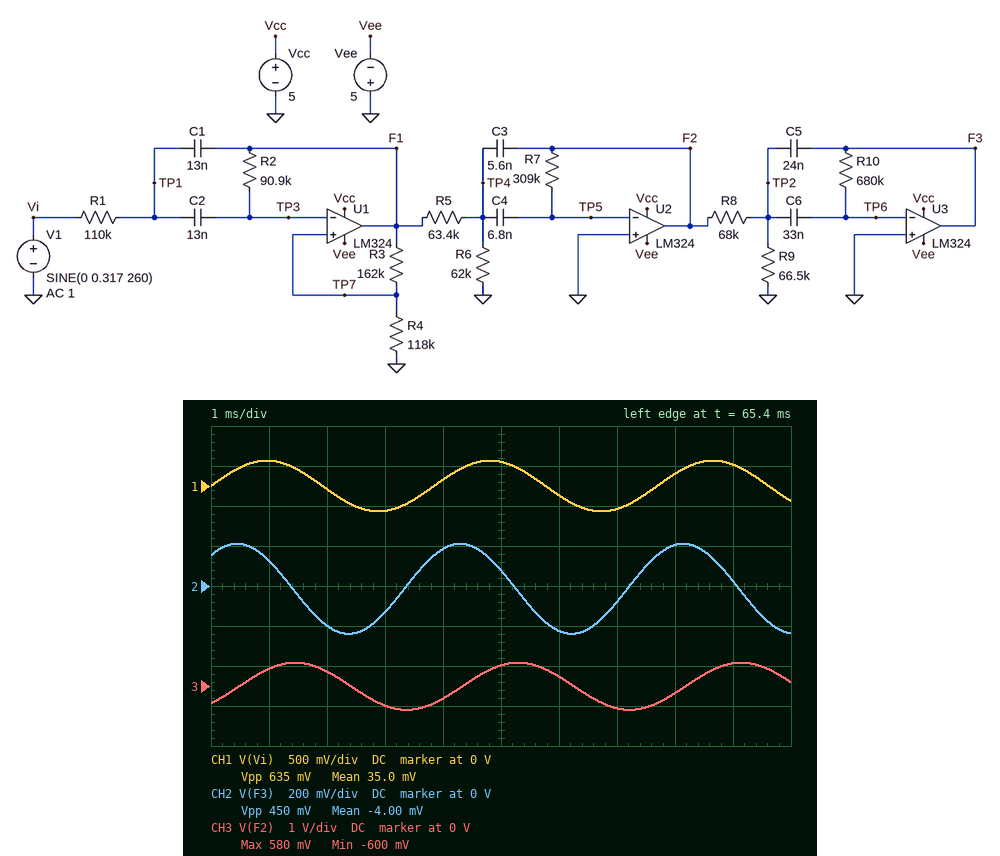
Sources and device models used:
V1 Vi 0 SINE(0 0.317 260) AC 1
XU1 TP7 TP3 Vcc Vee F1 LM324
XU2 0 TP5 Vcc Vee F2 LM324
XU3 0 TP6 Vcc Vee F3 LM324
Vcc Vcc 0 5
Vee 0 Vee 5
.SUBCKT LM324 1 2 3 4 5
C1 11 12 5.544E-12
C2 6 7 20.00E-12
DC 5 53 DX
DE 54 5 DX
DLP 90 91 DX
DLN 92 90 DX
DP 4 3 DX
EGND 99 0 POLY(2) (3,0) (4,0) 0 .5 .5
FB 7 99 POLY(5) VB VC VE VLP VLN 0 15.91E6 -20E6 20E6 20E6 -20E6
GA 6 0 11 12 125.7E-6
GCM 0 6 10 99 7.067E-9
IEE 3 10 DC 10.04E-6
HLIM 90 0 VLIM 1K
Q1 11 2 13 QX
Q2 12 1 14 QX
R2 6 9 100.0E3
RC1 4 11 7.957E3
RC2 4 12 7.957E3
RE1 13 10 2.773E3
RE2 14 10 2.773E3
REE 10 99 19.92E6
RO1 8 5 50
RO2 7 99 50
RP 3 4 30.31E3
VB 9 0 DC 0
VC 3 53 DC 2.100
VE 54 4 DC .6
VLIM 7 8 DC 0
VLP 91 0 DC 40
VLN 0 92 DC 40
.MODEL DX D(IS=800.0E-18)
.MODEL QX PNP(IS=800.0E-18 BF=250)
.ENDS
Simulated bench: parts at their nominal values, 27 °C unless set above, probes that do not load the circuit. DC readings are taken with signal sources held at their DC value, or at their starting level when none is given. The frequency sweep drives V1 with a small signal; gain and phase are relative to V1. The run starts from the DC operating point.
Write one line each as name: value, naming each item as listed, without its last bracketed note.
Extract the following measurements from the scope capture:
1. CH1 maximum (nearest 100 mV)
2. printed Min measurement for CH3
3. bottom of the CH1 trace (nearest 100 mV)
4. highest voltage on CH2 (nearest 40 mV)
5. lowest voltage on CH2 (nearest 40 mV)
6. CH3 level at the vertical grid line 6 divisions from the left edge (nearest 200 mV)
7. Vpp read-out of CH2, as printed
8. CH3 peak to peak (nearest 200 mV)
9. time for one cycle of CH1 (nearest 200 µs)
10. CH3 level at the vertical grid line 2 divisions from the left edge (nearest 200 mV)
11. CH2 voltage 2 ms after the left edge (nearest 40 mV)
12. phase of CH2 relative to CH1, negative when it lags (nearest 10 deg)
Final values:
CH1 maximum: 300 mV
printed Min measurement for CH3: -600 mV
bottom of the CH1 trace: -300 mV
highest voltage on CH2: 200 mV
lowest voltage on CH2: -240 mV
CH3 level at the vertical grid line 6 divisions from the left edge: 200 mV
Vpp read-out of CH2, as printed: 450 mV
CH3 peak to peak: 1.2 V
time for one cycle of CH1: 3.8 ms
CH3 level at the vertical grid line 2 divisions from the left edge: 400 mV
CH2 voltage 2 ms after the left edge: -200 mV
phase of CH2 relative to CH1, negative when it lags: 50 deg
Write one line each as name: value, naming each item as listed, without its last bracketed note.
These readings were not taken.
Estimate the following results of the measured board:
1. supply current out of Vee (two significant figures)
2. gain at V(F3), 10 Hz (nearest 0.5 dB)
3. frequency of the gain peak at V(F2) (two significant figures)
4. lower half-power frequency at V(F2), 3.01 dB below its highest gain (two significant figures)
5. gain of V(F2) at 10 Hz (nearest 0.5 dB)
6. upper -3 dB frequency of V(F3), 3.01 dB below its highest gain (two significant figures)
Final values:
supply current out of Vee: 1.0 mA
gain at V(F3), 10 Hz: -44.0 dB
frequency of the gain peak at V(F2): 240 Hz
lower half-power frequency at V(F2), 3.01 dB below its highest gain: 160 Hz
gain of V(F2) at 10 Hz: -41.5 dB
upper -3 dB frequency of V(F3), 3.01 dB below its highest gain: 280 Hz
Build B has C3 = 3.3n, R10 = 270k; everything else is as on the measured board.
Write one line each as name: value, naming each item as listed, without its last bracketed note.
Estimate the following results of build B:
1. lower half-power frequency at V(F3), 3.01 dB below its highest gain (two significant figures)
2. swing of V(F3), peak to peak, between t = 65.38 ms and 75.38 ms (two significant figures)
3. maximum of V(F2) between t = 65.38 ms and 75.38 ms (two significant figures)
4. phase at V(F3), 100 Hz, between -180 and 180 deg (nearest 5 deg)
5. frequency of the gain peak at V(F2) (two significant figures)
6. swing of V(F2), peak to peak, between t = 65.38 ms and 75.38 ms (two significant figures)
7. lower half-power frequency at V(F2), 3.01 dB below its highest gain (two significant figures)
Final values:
lower half-power frequency at V(F3), 3.01 dB below its highest gain: 58 Hz
swing of V(F3), peak to peak, between t = 65.38 ms and 75.38 ms: 440 mV
maximum of V(F2) between t = 65.38 ms and 75.38 ms: 560 mV
phase at V(F3), 100 Hz, between -180 and 180 deg: -145 deg
frequency of the gain peak at V(F2): 300 Hz
swing of V(F2), peak to peak, between t = 65.38 ms and 75.38 ms: 1.1 V
lower half-power frequency at V(F2), 3.01 dB below its highest gain: 180 Hz
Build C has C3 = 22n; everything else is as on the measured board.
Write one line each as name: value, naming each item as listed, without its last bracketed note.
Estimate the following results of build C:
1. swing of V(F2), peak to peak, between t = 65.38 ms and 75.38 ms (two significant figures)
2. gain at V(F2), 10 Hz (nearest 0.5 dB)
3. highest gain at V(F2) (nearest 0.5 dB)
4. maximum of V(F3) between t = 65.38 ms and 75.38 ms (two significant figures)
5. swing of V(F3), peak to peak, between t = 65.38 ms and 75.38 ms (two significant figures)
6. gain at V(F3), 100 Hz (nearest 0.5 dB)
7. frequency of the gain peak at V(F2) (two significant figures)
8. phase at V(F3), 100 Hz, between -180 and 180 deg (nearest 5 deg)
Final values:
swing of V(F2), peak to peak, between t = 65.38 ms and 75.38 ms: 230 mV
gain at V(F2), 10 Hz: -41.5 dB
highest gain at V(F2): 1.5 dB
maximum of V(F3) between t = 65.38 ms and 75.38 ms: 31 mV
swing of V(F3), peak to peak, between t = 65.38 ms and 75.38 ms: 89 mV
gain at V(F3), 100 Hz: 0 dB
frequency of the gain peak at V(F2): 130 Hz
phase at V(F3), 100 Hz, between -180 and 180 deg: 155 deg
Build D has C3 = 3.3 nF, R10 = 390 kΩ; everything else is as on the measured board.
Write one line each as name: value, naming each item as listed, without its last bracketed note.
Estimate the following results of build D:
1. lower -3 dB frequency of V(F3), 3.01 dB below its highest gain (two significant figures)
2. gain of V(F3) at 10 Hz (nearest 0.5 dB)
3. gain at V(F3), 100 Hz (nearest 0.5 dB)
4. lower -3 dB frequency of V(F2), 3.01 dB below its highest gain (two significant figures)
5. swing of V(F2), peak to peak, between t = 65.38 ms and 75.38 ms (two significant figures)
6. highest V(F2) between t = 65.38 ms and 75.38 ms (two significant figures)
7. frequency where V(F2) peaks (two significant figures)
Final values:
lower -3 dB frequency of V(F3), 3.01 dB below its highest gain: 47 Hz
gain of V(F3) at 10 Hz: -49.0 dB
gain at V(F3), 100 Hz: -1.5 dB
lower -3 dB frequency of V(F2), 3.01 dB below its highest gain: 180 Hz
swing of V(F2), peak to peak, between t = 65.38 ms and 75.38 ms: 1.1 V
highest V(F2) between t = 65.38 ms and 75.38 ms: 560 mV
frequency where V(F2) peaks: 300 Hz
